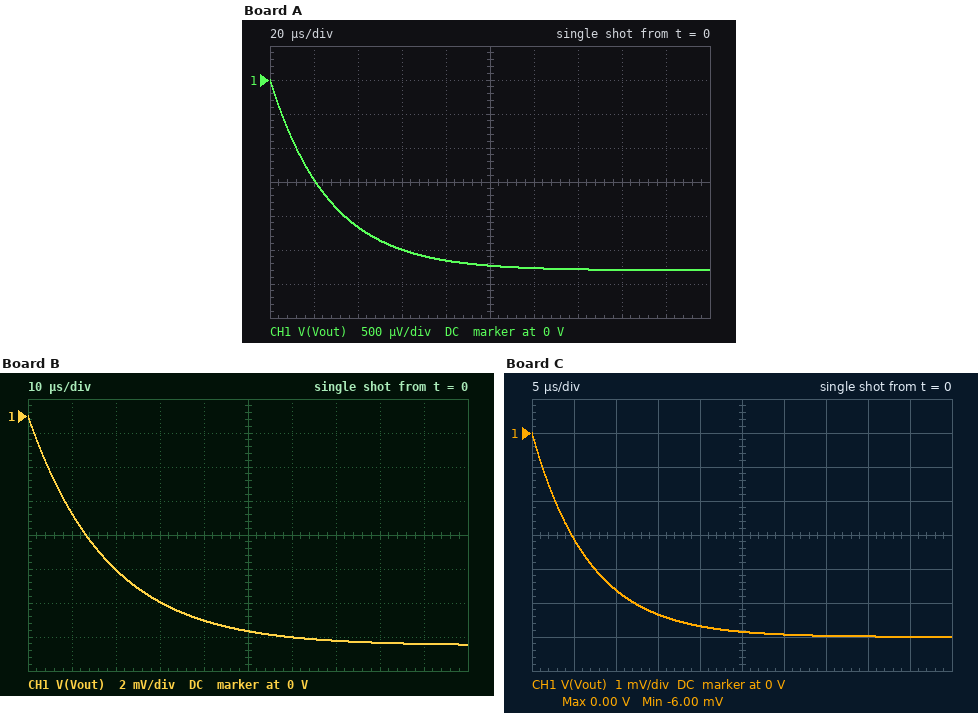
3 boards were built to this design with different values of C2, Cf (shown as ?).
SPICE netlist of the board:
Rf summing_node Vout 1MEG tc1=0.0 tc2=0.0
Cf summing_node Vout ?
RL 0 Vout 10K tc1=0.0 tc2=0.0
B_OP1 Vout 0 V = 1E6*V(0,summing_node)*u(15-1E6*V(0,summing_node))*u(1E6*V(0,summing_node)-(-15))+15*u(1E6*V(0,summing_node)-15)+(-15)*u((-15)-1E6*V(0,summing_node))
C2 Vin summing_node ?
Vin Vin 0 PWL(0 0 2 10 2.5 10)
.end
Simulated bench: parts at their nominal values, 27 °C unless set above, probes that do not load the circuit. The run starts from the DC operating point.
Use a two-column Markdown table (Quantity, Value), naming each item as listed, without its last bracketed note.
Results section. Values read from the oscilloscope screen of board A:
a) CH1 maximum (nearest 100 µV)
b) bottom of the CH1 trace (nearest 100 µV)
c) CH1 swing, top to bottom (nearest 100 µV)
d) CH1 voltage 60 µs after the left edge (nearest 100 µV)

| Quantity | Value |
|---|---|
| CH1 maximum | 0 V |
| bottom of the CH1 trace | -2.8 mV |
| CH1 swing, top to bottom | 2.8 mV |
| CH1 voltage 60 µs after the left edge | -2.5 mV |
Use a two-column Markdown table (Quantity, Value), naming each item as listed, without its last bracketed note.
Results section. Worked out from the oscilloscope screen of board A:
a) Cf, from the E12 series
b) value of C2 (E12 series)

| Quantity | Value |
|---|---|
| Cf, from the E12 series | 27 pF |
| value of C2 | 560 pF |
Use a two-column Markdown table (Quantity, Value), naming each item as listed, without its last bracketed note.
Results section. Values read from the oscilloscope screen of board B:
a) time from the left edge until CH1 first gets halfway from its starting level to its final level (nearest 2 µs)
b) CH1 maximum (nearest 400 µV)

| Quantity | Value |
|---|---|
| time from the left edge until CH1 first gets halfway from its starting level to its final level | 12 µs |
| CH1 maximum | 0 V |
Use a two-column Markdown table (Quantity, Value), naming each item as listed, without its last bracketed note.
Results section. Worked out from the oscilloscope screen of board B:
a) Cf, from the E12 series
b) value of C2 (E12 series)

| Quantity | Value |
|---|---|
| Cf, from the E12 series | 18 pF |
| value of C2 | 2.7 nF |
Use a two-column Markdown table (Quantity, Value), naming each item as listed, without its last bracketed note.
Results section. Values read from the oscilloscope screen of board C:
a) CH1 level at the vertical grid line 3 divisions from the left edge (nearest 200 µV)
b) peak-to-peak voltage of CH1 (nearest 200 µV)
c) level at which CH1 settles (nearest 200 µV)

| Quantity | Value |
|---|---|
| CH1 level at the vertical grid line 3 divisions from the left edge | -5.4 mV |
| peak-to-peak voltage of CH1 | 6.0 mV |
| level at which CH1 settles | -6.0 mV |
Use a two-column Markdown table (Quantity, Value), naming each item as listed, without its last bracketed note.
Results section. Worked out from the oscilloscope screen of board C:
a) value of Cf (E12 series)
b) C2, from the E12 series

| Quantity | Value |
|---|---|
| value of Cf | 6.8 pF |
| C2, from the E12 series | 1.2 nF |
